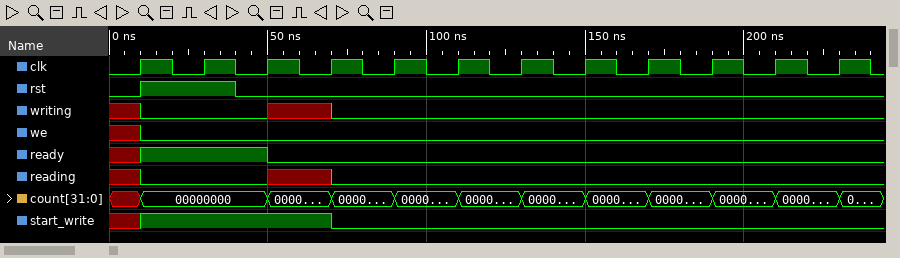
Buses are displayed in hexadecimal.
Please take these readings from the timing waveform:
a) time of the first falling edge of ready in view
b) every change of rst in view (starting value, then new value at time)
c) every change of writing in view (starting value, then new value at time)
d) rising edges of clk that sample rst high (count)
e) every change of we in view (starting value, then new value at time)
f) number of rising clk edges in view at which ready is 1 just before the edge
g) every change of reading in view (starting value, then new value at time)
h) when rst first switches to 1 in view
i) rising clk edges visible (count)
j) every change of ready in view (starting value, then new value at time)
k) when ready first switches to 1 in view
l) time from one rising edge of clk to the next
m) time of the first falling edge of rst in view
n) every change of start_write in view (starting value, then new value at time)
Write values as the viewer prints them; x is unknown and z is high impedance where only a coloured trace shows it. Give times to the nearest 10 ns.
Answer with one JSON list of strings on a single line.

["50 ns", "0, 1 at 10 ns, 0 at 40 ns", "x, 0 at 10 ns, x at 50 ns, 0 at 70 ns", "1", "x, 0 at 10 ns", "2", "x, 0 at 10 ns, x at 50 ns, 0 at 70 ns", "10 ns", "12", "x, 1 at 10 ns, 0 at 50 ns", "10 ns", "20 ns", "40 ns", "x, 1 at 10 ns, 0 at 70 ns"]
